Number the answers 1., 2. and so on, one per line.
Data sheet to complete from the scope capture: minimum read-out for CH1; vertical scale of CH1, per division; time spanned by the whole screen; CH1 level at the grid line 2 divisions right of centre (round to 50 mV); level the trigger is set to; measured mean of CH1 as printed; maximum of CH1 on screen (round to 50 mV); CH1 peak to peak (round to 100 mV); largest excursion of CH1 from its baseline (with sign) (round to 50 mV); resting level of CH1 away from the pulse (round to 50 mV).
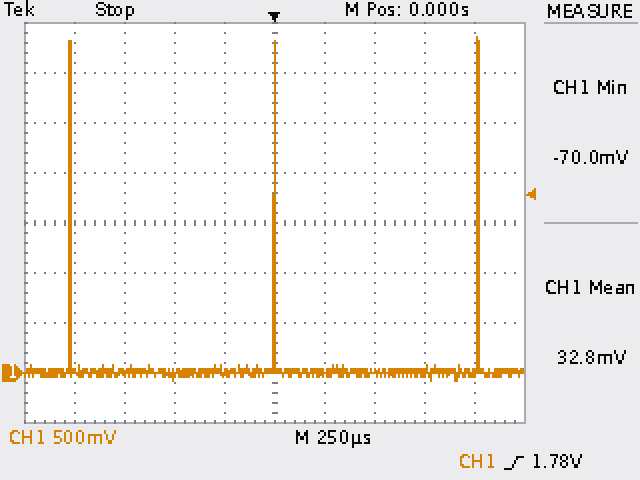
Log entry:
1. -70.0 mV
2. 500 mV
3. 2.5 ms
4. 0 mV
5. 1.78 V
6. 32.8 mV
7. 3.35 V
8. 3.40 V
9. +3.35 V
10. 0 mV
